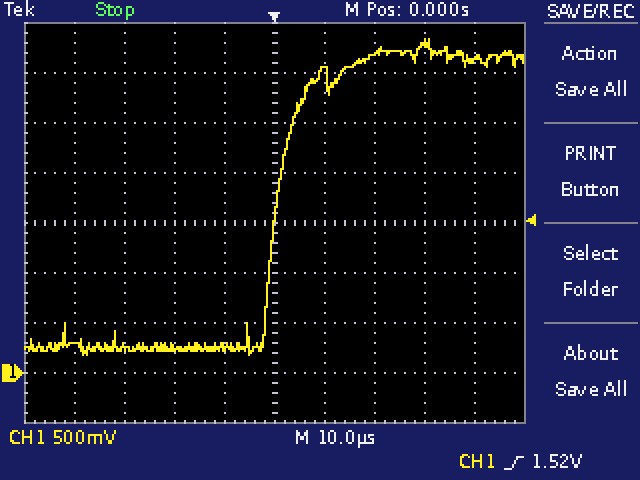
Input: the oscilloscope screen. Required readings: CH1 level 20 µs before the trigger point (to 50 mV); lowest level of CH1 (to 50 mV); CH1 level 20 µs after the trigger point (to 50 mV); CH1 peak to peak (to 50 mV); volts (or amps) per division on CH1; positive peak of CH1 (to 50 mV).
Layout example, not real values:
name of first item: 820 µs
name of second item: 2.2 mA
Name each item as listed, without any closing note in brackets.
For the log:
CH1 level 20 µs before the trigger point: 250 mV
lowest level of CH1: 200 mV
CH1 level 20 µs after the trigger point: 3.20 V
CH1 peak to peak: 3.15 V
volts (or amps) per division on CH1: 500 mV
positive peak of CH1: 3.35 V
